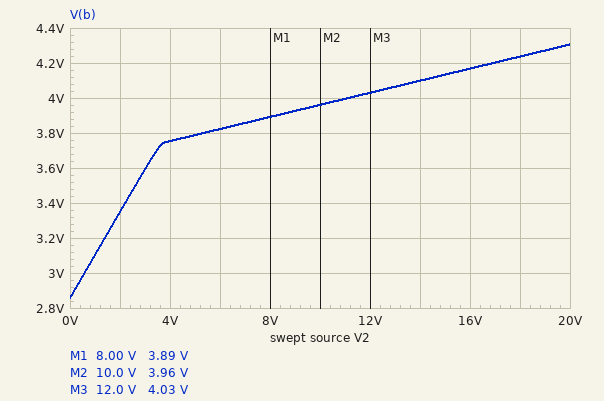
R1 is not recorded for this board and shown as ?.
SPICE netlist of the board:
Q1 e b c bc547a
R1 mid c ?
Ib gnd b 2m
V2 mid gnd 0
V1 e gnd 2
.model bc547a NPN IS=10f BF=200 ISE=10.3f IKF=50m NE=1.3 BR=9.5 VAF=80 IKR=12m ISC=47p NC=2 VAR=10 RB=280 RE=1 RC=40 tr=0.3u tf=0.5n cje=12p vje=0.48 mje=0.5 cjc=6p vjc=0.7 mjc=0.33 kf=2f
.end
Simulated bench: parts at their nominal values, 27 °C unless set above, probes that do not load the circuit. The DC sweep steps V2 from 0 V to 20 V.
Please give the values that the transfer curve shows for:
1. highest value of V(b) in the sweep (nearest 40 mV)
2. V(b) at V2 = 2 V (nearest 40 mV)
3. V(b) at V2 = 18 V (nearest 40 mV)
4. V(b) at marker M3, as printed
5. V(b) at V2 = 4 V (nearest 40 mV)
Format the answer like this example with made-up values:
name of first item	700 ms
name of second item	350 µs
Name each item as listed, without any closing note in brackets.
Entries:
highest value of V(b) in the sweep	4.32 V
V(b) at V2 = 2 V	3.36 V
V(b) at V2 = 18 V	4.24 V
V(b) at marker M3, as printed	4.03 V
V(b) at V2 = 4 V	3.76 V
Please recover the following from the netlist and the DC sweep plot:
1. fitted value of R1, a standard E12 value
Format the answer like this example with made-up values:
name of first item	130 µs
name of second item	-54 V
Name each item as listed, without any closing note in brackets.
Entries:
fitted value of R1, a standard E12 value	120 Ω
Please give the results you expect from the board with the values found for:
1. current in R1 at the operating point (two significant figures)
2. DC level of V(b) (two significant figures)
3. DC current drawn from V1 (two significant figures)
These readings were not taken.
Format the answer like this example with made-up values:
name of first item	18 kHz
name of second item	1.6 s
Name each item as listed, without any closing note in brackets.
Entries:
current in R1 at the operating point	13 mA
DC level of V(b)	2.9 V
DC current drawn from V1	11 mA
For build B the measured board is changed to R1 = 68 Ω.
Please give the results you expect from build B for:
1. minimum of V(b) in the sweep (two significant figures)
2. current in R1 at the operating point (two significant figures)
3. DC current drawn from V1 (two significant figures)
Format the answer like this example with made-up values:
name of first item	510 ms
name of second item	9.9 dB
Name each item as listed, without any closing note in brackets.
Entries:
minimum of V(b) in the sweep	2.6 V
current in R1 at the operating point	19 mA
DC current drawn from V1	17 mA
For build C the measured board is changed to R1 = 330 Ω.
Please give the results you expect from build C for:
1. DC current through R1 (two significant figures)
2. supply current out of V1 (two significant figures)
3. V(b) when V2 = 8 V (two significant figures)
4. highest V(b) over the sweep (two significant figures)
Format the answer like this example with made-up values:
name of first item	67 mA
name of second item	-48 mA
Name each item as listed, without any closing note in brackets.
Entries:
DC current through R1	5.6 mA
supply current out of V1	3.6 mA
V(b) when V2 = 8 V	3.8 V
highest V(b) over the sweep	4.2 V
